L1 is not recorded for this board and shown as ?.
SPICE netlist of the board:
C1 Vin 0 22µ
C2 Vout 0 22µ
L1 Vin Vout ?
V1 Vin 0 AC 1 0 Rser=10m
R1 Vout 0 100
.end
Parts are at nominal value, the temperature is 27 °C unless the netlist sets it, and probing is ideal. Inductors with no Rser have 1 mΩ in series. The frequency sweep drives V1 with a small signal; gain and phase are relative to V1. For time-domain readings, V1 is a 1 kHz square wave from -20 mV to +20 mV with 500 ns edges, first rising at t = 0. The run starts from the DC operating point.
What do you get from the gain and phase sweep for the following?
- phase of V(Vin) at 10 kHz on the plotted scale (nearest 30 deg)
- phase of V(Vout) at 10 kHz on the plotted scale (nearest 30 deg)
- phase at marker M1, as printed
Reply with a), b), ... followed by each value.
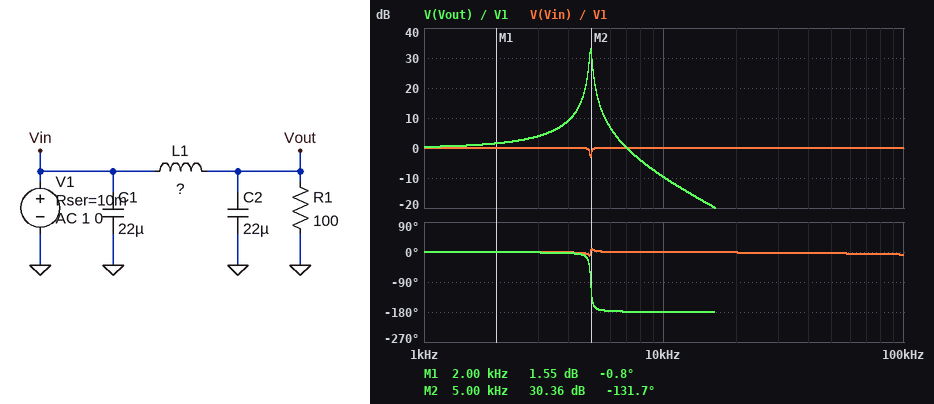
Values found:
a) 0 deg
b) -180 deg
c) -0.8 deg
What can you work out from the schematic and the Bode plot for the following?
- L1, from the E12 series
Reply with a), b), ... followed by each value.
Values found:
a) 47 µH
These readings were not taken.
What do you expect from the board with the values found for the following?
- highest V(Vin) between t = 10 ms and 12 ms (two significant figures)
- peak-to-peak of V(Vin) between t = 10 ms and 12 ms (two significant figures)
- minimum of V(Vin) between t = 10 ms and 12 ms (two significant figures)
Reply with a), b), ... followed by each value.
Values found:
a) 21 mV
b) 42 mV
c) -21 mV
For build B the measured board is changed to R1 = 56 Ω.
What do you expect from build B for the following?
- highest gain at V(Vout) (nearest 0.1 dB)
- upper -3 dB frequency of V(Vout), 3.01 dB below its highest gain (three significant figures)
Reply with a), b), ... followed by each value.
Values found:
a) 29.5 dB
b) 5.03 kHz
